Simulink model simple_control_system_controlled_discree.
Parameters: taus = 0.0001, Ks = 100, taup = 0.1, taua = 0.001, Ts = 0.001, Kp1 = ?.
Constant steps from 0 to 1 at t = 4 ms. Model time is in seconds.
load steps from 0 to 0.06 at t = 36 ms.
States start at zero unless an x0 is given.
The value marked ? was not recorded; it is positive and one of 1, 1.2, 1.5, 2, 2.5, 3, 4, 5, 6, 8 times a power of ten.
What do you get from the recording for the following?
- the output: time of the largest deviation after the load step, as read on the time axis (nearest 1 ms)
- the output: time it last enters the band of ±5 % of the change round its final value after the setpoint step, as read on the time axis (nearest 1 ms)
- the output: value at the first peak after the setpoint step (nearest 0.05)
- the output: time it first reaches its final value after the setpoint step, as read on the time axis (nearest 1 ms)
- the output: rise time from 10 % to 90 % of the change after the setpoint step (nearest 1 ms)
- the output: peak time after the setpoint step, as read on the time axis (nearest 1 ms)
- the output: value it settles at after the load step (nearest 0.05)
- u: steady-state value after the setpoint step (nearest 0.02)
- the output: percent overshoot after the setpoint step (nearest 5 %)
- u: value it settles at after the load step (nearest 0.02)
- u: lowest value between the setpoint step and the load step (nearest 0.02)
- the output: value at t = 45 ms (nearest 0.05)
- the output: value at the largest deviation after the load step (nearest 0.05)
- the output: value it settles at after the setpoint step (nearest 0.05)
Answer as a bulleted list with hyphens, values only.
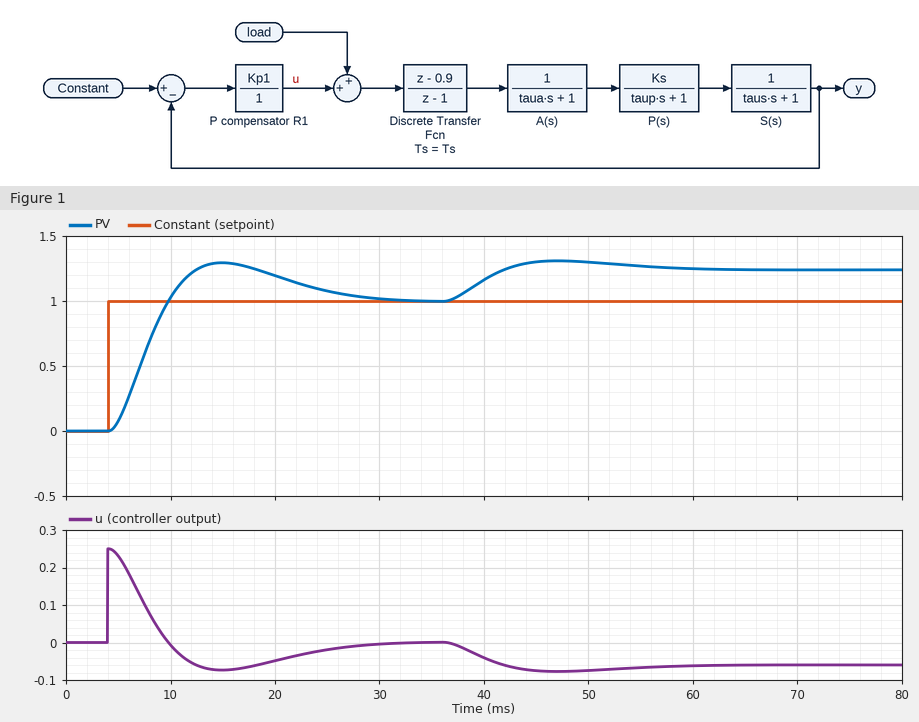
- 47 ms
- 27 ms
- 1.30
- 10 ms
- 4 ms
- 15 ms
- 1.25
- 0.00
- 30 %
- -0.06
- -0.08
- 1.30
- 1.30
- 1.00
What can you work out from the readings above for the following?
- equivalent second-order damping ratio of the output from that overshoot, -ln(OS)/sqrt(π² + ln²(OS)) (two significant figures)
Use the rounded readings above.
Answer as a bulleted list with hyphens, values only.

- 0.36
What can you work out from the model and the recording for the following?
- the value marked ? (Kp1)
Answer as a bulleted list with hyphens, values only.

- 0.25
